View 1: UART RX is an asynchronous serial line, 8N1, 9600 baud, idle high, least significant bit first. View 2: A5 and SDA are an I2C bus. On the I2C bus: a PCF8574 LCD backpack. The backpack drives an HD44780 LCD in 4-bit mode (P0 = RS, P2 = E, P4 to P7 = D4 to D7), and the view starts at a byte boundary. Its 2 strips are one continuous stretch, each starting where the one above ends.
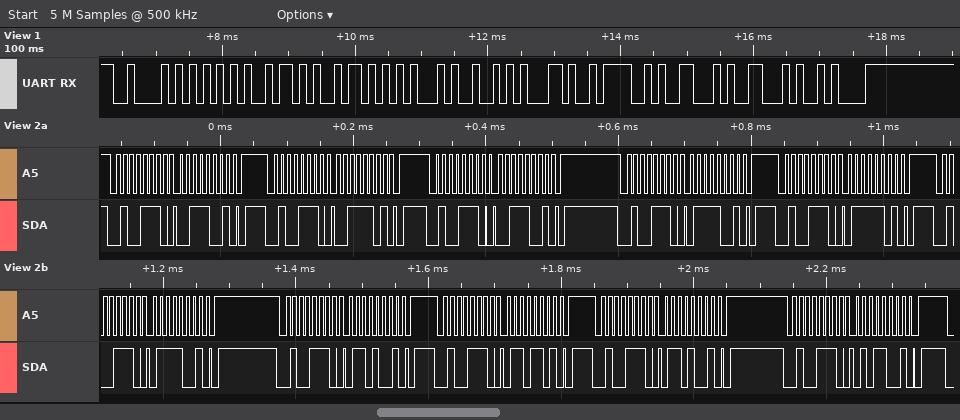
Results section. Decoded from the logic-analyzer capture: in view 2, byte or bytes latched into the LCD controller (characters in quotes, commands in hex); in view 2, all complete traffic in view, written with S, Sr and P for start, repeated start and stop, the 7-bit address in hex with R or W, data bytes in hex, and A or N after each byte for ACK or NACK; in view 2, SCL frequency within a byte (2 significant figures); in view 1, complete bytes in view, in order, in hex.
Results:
'7'
S 27W A 39 A P S 27W A 3D A P S 27W A 39 A P S 27W A 79 A P S 27W A 7D A P S 27W A 79 A P S 27W A 69 A P S 27W A 6D A P S 27W A 69 A P S 27W A 59 A P
100 kHz
0x42 0x55 0x5A 0x5A 0x45 0x52 0x2C 0x4F 0x46 0x46 0x0A
